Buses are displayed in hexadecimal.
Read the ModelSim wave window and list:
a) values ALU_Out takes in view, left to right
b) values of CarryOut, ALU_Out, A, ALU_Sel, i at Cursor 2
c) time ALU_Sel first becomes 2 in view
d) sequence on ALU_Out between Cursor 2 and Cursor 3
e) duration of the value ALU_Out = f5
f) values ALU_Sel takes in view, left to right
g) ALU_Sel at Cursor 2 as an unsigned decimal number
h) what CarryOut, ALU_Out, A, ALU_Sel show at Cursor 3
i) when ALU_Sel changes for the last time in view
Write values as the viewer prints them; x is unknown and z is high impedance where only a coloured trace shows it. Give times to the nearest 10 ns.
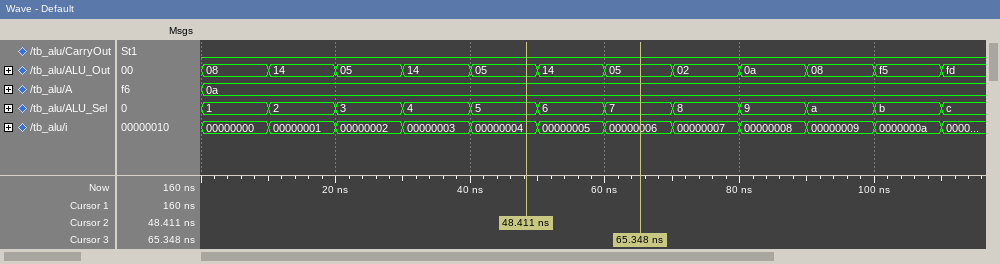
08, 14, 05, 14, 05, 14, 05, 02, 0a, 08, f5, fd
CarryOut=0, ALU_Out=05, A=0a, ALU_Sel=5, i=00000004
10 ns
05, 14, 05
10 ns
1, 2, 3, 4, 5, 6, 7, 8, 9, a, b, c
5
CarryOut=0, ALU_Out=05, A=0a, ALU_Sel=7
110 ns
